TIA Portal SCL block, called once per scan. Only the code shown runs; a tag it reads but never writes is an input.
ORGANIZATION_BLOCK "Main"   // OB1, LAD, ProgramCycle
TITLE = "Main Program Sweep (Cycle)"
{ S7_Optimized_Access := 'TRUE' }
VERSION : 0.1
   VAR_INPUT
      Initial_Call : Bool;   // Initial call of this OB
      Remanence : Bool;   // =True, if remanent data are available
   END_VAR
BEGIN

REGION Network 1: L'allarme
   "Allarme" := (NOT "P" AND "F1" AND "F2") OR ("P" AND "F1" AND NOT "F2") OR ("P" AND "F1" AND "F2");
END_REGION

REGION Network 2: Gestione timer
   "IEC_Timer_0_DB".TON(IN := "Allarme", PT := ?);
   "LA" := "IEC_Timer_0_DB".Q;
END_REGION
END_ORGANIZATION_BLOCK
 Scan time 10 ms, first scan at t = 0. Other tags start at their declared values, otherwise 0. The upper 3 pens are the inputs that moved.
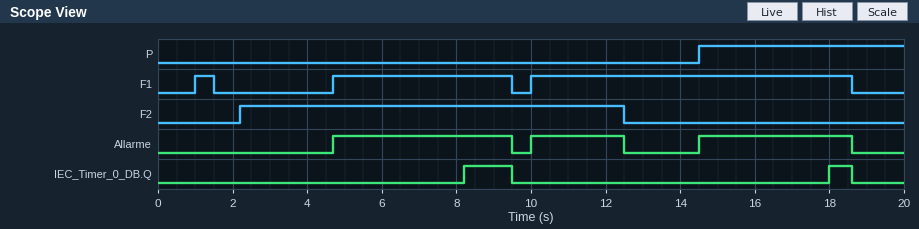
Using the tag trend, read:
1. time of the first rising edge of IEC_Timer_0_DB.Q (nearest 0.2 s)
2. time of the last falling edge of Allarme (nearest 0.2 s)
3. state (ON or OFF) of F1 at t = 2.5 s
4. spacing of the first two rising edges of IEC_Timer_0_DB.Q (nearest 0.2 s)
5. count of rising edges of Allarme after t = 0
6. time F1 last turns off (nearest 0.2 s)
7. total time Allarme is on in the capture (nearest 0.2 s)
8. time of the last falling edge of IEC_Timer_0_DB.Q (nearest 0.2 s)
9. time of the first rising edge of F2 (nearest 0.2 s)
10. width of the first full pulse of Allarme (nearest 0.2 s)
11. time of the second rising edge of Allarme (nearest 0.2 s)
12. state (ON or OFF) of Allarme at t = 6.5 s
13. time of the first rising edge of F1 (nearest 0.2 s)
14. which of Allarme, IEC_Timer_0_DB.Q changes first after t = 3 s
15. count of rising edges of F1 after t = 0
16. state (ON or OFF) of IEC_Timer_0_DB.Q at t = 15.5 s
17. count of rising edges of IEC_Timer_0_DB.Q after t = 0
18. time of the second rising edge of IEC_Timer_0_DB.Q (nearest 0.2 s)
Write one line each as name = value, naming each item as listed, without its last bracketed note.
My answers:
time of the first rising edge of IEC_Timer_0_DB.Q = 8.2 s
time of the last falling edge of Allarme = 18.6 s
state (ON or OFF) of F1 at t = 2.5 s = OFF
spacing of the first two rising edges of IEC_Timer_0_DB.Q = 9.8 s
count of rising edges of Allarme after t = 0 = 3
time F1 last turns off = 18.6 s
total time Allarme is on in the capture = 11.4 s
time of the last falling edge of IEC_Timer_0_DB.Q = 18.6 s
time of the first rising edge of F2 = 2.2 s
width of the first full pulse of Allarme = 4.8 s
time of the second rising edge of Allarme = 10.0 s
state (ON or OFF) of Allarme at t = 6.5 s = ON
time of the first rising edge of F1 = 1.0 s
which of Allarme, IEC_Timer_0_DB.Q changes first after t = 3 s = Allarme
count of rising edges of F1 after t = 0 = 3
state (ON or OFF) of IEC_Timer_0_DB.Q at t = 15.5 s = OFF
count of rising edges of IEC_Timer_0_DB.Q after t = 0 = 2
time of the second rising edge of IEC_Timer_0_DB.Q = 18.0 s
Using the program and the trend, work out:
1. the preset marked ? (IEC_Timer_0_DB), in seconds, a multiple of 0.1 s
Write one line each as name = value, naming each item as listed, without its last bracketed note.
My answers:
the preset marked ? (IEC_Timer_0_DB), in seconds, a multiple of 0.1 s = 3.5 s
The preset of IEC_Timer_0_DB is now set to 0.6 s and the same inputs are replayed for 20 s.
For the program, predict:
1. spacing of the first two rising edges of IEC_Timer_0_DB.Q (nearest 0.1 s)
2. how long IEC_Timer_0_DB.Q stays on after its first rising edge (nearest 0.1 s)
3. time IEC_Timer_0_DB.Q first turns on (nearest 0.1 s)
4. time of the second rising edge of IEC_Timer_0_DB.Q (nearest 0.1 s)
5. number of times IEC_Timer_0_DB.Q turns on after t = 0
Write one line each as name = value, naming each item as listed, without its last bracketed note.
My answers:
spacing of the first two rising edges of IEC_Timer_0_DB.Q = 5.3 s
how long IEC_Timer_0_DB.Q stays on after its first rising edge = 4.2 s
time IEC_Timer_0_DB.Q first turns on = 5.3 s
time of the second rising edge of IEC_Timer_0_DB.Q = 10.6 s
number of times IEC_Timer_0_DB.Q turns on after t = 0 = 3
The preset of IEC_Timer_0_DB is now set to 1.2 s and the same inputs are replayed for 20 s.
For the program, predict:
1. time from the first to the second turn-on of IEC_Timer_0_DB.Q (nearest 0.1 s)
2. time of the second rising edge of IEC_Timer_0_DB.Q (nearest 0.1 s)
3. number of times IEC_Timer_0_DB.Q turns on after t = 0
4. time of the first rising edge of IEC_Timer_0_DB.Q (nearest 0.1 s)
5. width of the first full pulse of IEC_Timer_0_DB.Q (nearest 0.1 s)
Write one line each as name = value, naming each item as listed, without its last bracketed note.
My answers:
time from the first to the second turn-on of IEC_Timer_0_DB.Q = 5.3 s
time of the second rising edge of IEC_Timer_0_DB.Q = 11.2 s
number of times IEC_Timer_0_DB.Q turns on after t = 0 = 3
time of the first rising edge of IEC_Timer_0_DB.Q = 5.9 s
width of the first full pulse of IEC_Timer_0_DB.Q = 3.6 s
